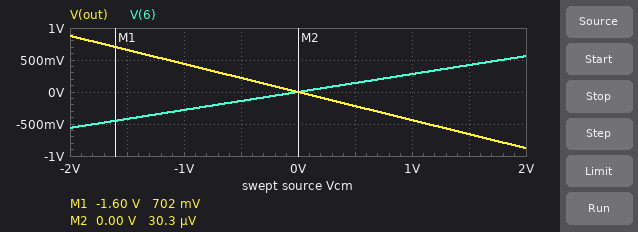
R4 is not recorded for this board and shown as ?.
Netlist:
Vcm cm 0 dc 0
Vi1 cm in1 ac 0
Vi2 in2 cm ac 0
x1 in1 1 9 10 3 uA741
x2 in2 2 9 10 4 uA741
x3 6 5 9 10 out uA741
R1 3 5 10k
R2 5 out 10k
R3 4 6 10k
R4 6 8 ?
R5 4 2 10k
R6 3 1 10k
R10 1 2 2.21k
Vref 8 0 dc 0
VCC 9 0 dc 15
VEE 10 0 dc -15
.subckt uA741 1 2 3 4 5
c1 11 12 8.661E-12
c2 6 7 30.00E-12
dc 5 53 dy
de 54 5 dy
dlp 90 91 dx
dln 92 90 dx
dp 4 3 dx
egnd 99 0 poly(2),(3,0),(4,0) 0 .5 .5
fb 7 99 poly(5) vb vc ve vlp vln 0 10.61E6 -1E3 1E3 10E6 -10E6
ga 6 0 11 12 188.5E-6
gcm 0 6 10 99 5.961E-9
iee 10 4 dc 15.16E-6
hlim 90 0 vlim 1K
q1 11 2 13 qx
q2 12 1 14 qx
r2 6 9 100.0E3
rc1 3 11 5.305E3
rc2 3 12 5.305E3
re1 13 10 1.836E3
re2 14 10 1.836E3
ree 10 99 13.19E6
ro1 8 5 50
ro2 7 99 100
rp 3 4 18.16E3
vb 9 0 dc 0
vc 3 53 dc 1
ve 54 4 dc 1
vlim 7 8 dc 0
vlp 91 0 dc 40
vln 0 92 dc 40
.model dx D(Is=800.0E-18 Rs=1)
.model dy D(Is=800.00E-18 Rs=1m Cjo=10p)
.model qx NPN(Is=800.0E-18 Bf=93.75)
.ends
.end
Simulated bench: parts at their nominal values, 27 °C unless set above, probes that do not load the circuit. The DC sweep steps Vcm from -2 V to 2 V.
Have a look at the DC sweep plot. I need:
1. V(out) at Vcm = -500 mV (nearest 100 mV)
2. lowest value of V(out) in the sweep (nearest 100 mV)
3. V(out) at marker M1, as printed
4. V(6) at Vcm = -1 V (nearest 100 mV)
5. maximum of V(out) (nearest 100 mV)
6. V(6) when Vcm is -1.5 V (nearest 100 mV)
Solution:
200 mV
-900 mV
702 mV
-300 mV
900 mV
-400 mV
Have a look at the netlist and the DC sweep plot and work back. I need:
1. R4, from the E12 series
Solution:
3.9 kΩ
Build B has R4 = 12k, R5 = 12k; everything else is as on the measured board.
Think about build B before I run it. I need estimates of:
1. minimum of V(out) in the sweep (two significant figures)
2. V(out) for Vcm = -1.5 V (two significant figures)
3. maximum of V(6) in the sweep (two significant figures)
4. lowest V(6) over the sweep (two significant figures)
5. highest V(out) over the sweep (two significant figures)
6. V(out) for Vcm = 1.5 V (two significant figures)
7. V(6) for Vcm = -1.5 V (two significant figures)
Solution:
-180 mV
-140 mV
1.1 V
-1.1 V
180 mV
140 mV
-820 mV
